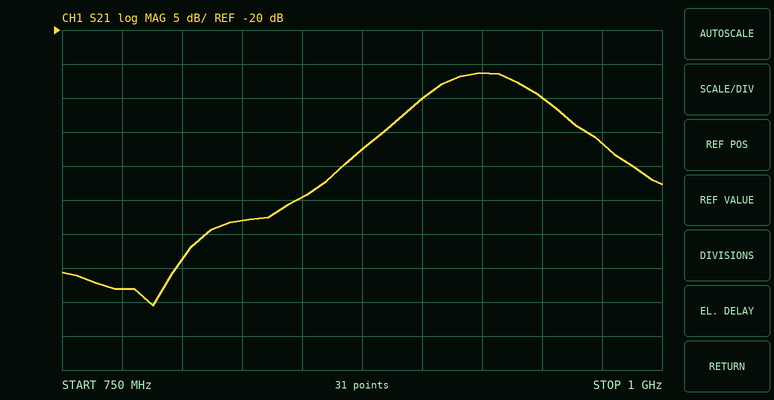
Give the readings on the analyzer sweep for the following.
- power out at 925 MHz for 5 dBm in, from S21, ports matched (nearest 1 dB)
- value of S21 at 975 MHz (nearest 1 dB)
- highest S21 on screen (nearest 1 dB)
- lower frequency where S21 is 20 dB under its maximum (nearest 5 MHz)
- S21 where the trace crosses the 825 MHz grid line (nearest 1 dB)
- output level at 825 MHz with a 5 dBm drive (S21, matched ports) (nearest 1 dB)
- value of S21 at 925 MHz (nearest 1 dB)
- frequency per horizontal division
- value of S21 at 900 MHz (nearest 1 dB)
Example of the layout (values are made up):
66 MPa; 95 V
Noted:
-21 dBm; -37 dB; -26 dB; 840 MHz; -48 dB; -43 dBm; -26 dB; 25 MHz; -30 dB
